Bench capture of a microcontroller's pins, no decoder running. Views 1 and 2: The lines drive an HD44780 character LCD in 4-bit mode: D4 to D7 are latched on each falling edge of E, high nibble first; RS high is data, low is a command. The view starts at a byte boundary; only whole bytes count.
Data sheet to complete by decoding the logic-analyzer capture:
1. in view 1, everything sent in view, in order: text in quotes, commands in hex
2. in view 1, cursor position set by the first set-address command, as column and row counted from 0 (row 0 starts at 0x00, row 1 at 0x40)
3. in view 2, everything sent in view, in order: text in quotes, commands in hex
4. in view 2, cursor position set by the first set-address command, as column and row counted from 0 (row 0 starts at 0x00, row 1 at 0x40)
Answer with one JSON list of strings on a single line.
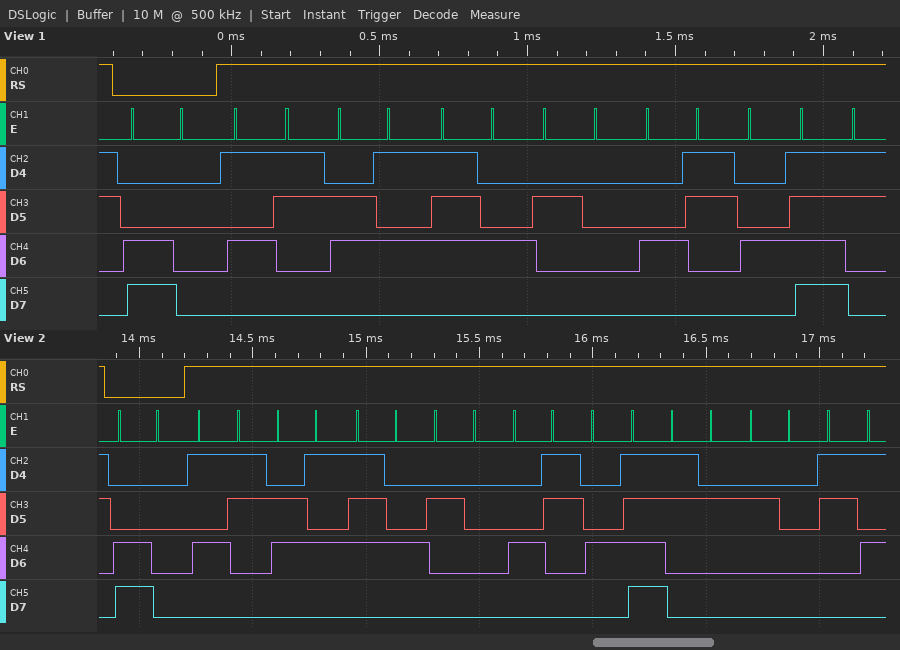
["0xC0 \"Set CO\"", "column 0, row 1", "0xC0 \"Set CO2 5\"", "column 0, row 1"]
